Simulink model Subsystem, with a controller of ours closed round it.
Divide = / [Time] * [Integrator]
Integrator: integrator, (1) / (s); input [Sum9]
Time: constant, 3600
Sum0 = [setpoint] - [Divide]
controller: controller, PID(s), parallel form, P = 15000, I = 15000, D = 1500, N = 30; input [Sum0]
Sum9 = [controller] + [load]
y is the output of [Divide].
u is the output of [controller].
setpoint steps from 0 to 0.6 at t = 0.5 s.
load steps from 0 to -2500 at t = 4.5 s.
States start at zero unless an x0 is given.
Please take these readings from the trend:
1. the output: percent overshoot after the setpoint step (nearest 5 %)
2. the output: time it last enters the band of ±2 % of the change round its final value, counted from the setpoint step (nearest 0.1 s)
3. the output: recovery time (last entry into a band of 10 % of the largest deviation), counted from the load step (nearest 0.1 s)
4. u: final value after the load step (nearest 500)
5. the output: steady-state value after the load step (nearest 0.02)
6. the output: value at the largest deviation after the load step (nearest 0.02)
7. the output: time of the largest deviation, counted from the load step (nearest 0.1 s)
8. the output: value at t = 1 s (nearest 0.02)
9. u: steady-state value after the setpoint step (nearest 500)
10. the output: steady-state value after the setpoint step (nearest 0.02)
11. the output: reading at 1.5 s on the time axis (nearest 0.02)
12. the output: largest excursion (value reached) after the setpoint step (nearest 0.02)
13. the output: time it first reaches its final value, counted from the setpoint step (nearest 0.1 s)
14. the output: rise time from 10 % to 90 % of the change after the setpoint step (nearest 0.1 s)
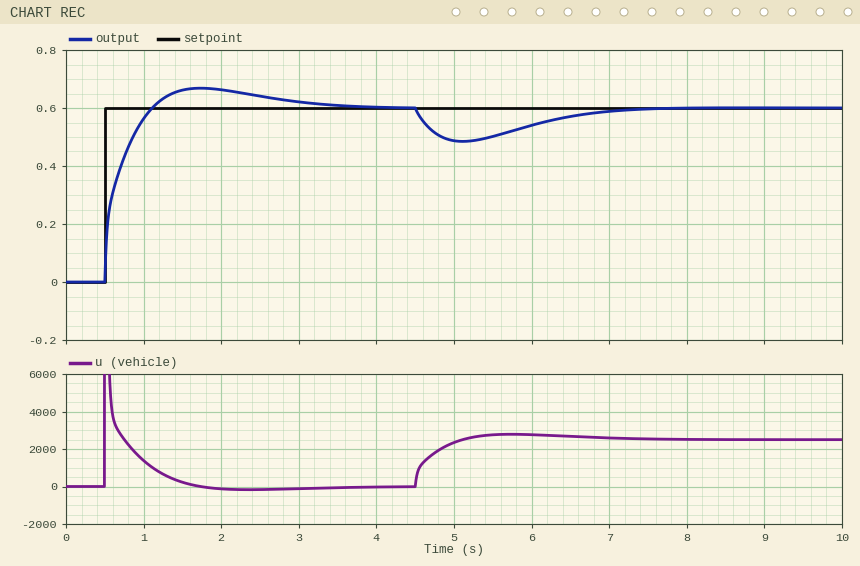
10 %
2.8 s
2.5 s
2500
0.60
0.48
0.6 s
0.56
0
0.60
0.66
0.66
0.6 s
0.4 s
